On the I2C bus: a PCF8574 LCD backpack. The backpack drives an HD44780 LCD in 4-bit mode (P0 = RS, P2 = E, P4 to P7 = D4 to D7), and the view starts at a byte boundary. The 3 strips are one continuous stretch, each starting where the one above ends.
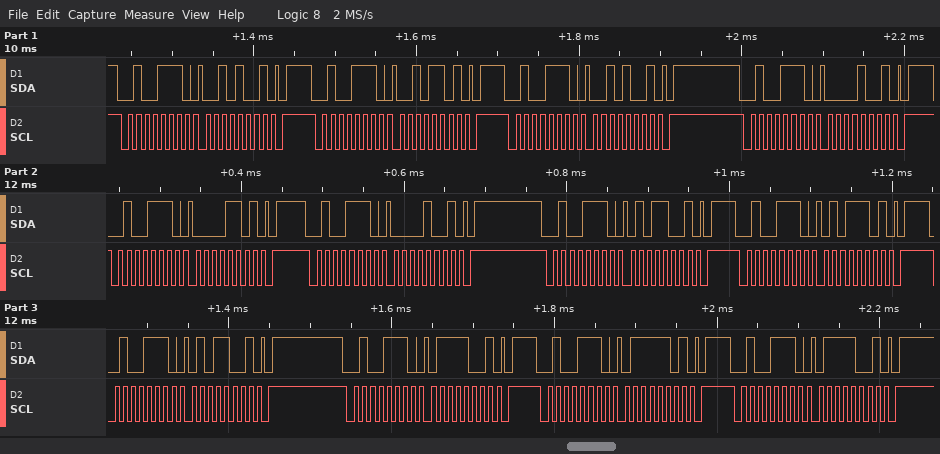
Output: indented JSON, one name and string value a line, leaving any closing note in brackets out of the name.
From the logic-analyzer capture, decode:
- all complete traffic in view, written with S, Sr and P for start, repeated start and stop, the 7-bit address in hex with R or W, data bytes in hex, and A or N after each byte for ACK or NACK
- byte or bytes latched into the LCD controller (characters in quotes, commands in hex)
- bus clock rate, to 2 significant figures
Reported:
{
  "all complete traffic in view, written with S, Sr and P for start, repeated start and stop, the 7-bit address in hex with R or W, data bytes in hex, and A or N after each byte for ACK or NACK": "S 27W A 29 A P S 27W A 2D A P S 27W A 29 A P S 27W A 09 A P S 27W A 0D A P S 27W A 09 A P S 27W A 59 A P S 27W A 5D A P S 27W A 59 A P S 27W A 79 A P S 27W A 7D A P S 27W A 79 A P",
  "byte or bytes latched into the LCD controller": "' ' 'W'",
  "bus clock rate, to 2 significant figures": "100 kHz"
}
